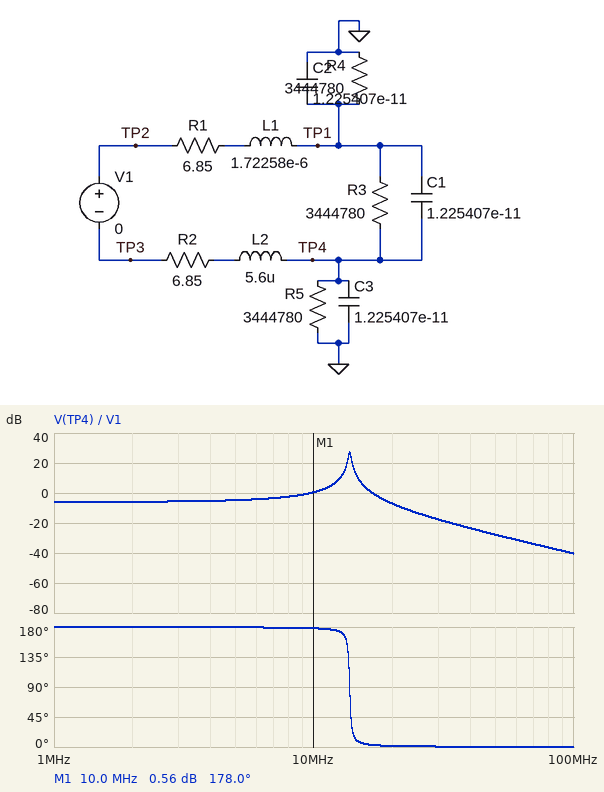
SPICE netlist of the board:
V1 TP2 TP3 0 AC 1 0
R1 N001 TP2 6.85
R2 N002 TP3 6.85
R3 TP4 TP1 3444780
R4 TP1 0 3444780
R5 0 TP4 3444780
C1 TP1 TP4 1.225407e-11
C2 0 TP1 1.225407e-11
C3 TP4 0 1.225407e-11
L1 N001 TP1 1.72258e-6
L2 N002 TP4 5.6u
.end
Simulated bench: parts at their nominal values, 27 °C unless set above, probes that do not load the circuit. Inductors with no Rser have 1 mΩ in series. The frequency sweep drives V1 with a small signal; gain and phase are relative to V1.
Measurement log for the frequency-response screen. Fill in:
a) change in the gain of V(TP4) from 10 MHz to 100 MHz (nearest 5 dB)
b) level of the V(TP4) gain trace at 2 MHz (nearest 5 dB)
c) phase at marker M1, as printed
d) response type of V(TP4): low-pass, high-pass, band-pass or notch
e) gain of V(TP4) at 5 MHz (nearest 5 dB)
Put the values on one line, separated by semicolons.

-40 dB; -5 dB; 178.0 deg; low-pass; -5 dB
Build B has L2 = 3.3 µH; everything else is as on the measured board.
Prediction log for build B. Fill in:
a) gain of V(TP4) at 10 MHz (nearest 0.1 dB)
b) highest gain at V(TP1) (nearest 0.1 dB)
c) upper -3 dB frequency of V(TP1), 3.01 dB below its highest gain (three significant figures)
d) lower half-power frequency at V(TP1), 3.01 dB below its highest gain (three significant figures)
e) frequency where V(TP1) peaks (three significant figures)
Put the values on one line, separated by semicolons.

-2.1 dB; 25.5 dB; 16.8 MHz; 16.3 MHz; 16.6 MHz
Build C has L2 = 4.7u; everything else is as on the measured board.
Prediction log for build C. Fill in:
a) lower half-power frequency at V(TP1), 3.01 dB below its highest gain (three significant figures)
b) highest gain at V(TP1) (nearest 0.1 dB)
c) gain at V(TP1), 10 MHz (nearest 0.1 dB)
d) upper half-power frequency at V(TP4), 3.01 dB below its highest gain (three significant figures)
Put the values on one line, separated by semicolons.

14.5 MHz; 26.6 dB; -0.6 dB; 14.8 MHz
